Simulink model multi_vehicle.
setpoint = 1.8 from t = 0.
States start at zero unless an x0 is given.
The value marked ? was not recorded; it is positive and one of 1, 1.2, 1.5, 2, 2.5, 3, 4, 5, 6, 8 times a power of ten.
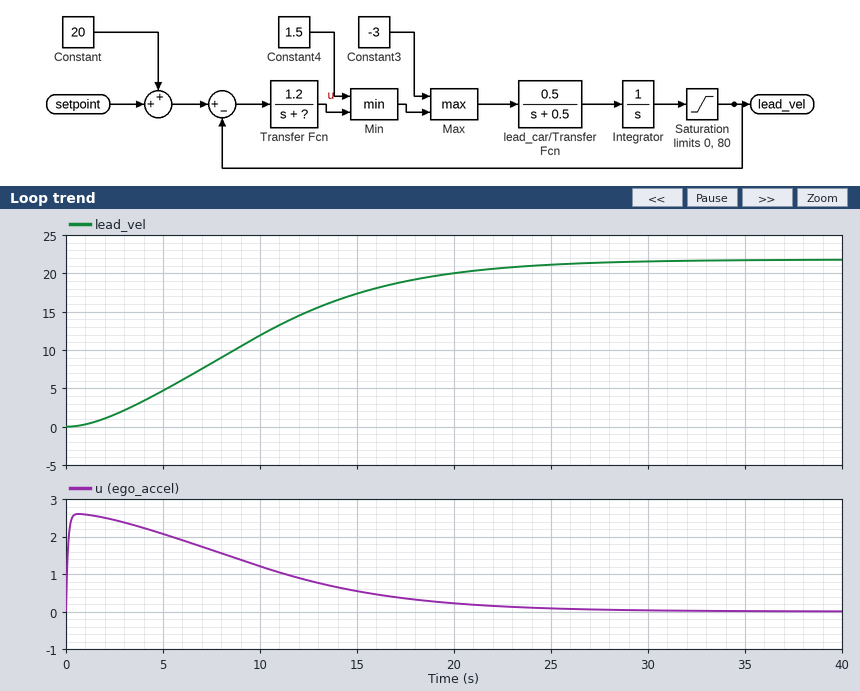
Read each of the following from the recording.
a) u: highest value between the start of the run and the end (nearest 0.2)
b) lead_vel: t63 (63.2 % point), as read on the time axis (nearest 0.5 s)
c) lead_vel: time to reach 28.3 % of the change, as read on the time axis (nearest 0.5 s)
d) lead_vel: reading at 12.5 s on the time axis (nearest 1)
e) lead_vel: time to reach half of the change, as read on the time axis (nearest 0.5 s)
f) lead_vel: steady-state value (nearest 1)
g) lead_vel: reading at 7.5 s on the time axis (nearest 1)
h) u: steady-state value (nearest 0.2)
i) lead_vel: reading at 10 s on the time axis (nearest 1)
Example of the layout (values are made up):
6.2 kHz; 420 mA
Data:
2.6; 11.5 s; 6.0 s; 15; 9.5 s; 22; 8; 0.0; 12
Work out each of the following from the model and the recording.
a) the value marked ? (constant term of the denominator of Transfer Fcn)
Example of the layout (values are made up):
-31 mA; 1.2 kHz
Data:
10
